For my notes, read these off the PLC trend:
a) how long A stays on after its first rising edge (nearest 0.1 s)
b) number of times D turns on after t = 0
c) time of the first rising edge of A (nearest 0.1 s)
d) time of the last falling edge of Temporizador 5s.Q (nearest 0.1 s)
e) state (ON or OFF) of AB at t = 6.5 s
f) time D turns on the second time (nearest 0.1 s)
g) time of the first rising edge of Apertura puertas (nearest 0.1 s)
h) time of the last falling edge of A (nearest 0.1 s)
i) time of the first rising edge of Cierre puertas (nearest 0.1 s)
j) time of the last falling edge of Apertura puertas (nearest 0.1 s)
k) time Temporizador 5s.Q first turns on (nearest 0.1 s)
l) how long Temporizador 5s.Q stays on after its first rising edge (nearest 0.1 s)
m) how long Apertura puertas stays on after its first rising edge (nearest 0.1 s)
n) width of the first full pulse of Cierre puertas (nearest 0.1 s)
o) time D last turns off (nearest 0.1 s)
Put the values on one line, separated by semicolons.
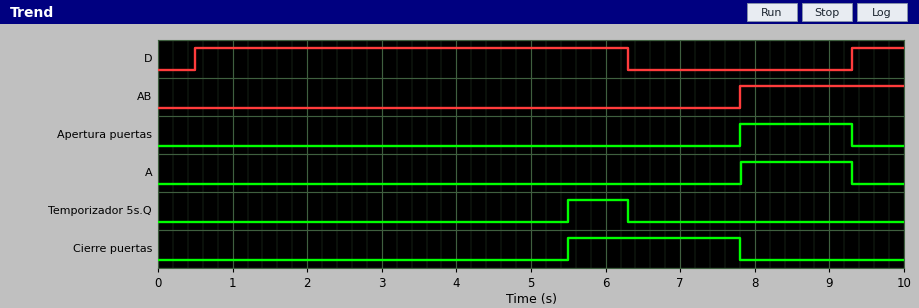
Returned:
1.5 s; 2; 7.8 s; 6.3 s; OFF; 9.3 s; 7.8 s; 9.3 s; 5.5 s; 9.3 s; 5.5 s; 0.8 s; 1.5 s; 2.3 s; 6.3 s
